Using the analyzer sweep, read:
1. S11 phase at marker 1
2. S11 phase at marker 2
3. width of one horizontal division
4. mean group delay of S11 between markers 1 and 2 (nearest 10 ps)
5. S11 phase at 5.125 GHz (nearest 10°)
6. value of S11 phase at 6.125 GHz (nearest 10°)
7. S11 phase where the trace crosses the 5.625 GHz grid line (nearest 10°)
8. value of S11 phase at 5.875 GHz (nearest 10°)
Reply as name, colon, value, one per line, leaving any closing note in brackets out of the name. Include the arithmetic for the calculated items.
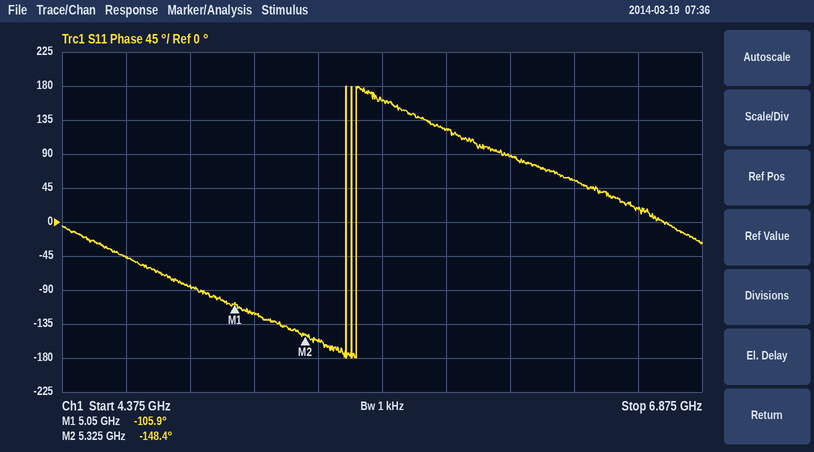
S11 phase at marker 1: -105.9°
S11 phase at marker 2: -148.4°
width of one horizontal division: 250 MHz
mean group delay of S11 between markers 1 and 2: −(-148.4° − (-105.9°))/(360° × 275 MHz) ≈ 429 ps, so 430 ps to the nearest 10 ps
S11 phase at 5.125 GHz: -120°
value of S11 phase at 6.125 GHz: 90°
S11 phase where the trace crosses the 5.625 GHz grid line: 160°
value of S11 phase at 5.875 GHz: 120°
